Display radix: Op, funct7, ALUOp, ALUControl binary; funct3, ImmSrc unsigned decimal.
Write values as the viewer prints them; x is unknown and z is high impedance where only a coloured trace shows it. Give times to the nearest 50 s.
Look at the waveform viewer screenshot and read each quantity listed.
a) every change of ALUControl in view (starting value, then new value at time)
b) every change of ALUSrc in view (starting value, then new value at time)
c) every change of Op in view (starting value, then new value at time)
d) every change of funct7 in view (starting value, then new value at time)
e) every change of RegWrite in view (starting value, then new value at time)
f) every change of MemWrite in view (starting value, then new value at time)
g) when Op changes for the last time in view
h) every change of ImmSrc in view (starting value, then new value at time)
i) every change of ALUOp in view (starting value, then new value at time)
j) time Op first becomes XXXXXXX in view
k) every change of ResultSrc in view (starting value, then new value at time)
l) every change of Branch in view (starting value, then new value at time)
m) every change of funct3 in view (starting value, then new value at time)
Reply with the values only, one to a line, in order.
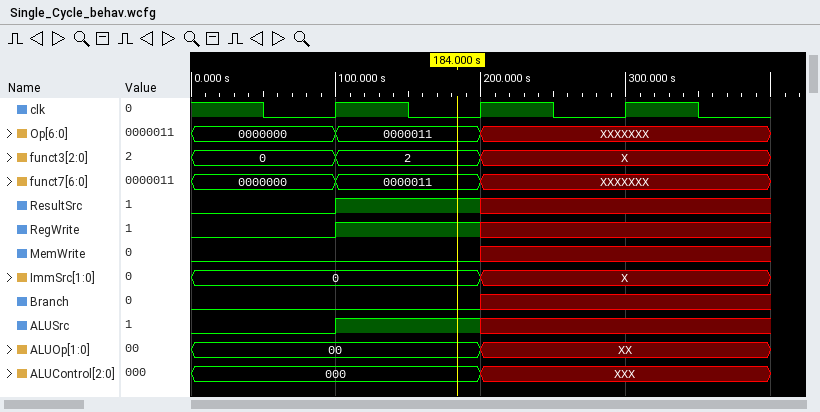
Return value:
000, XXX at 200 s
0, 1 at 100 s, x at 200 s
0000000, 0000011 at 100 s, XXXXXXX at 200 s
0000000, 0000011 at 100 s, XXXXXXX at 200 s
0, 1 at 100 s, x at 200 s
0, x at 200 s
200 s
0, X at 200 s
00, XX at 200 s
200 s
0, 1 at 100 s, x at 200 s
0, x at 200 s
0, 2 at 100 s, X at 200 s
